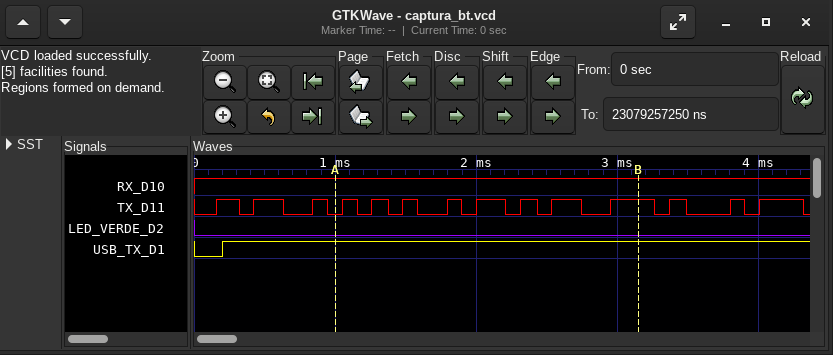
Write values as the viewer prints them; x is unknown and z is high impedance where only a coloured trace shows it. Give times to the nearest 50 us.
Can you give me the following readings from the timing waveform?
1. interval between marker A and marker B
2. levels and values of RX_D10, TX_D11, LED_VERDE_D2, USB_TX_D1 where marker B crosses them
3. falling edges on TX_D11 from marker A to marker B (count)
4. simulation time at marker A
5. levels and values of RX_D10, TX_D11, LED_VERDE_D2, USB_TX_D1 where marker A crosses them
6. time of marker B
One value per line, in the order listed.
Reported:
2150 us
RX_D10=1, TX_D11=1, LED_VERDE_D2=0, USB_TX_D1=1
7
1000 us
RX_D10=1, TX_D11=0, LED_VERDE_D2=0, USB_TX_D1=1
3150 us
